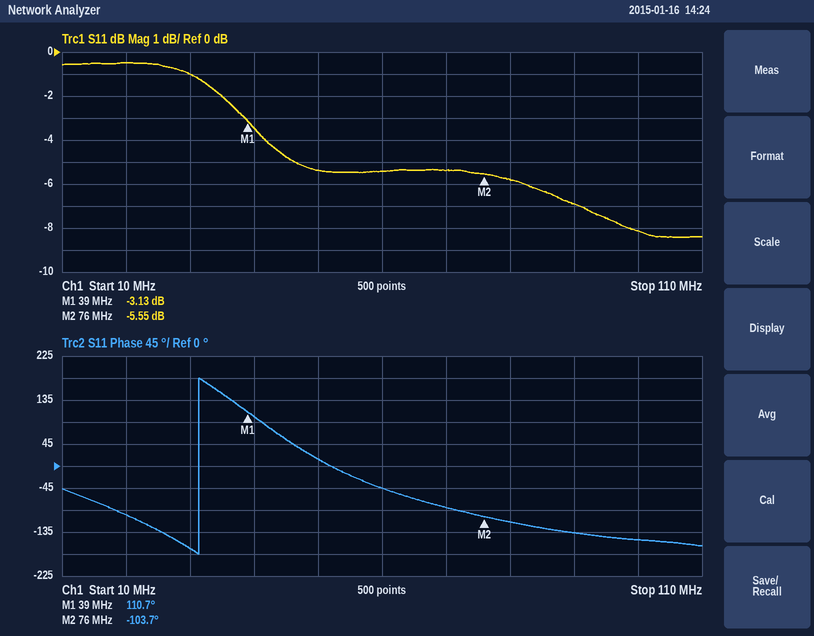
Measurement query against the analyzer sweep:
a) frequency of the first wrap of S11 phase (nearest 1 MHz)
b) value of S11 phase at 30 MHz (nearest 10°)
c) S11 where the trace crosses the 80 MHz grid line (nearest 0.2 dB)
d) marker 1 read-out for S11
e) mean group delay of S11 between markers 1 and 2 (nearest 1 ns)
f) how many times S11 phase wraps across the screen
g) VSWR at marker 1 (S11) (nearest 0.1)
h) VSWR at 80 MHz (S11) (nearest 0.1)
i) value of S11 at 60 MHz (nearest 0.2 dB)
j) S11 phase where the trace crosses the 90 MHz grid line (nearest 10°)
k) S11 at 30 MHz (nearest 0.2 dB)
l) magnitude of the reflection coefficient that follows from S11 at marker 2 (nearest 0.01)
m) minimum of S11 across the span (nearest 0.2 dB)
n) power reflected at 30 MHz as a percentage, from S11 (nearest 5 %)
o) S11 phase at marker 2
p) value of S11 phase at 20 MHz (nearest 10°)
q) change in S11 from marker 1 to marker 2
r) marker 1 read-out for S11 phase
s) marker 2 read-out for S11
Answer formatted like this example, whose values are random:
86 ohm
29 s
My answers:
31 MHz
-170°
-5.8 dB
-3.13 dB
16 ns
1
5.6
3.1
-5.4 dB
-140°
-1.0 dB
0.53
-8.4 dB
80 %
-103.7°
-100°
-2.42 dB
110.7°
-5.55 dB
